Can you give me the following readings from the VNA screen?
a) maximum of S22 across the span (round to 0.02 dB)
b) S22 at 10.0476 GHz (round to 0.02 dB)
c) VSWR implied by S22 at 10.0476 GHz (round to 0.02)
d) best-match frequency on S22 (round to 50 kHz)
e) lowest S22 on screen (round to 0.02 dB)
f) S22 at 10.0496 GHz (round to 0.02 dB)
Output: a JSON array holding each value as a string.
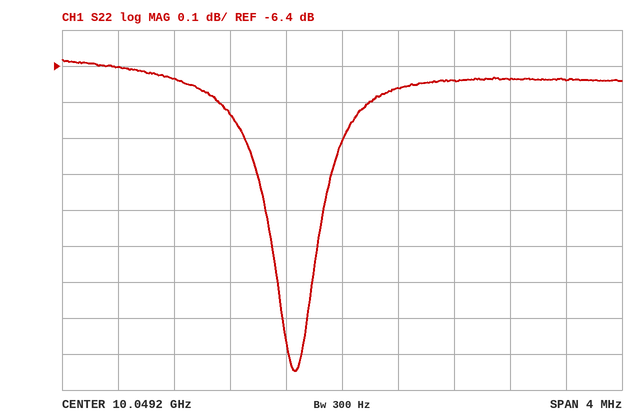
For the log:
["-6.38 dB", "-6.40 dB", "2.84", "10.04885 GHz", "-7.24 dB", "-6.46 dB"]
